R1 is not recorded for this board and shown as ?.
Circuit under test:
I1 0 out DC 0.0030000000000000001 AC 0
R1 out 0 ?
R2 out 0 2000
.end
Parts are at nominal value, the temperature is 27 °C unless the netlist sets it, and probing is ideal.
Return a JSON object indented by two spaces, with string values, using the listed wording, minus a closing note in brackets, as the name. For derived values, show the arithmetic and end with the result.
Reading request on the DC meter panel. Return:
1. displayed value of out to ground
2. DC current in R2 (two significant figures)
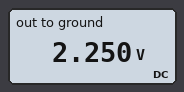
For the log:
{
  "displayed value of out to ground": "2.250 V",
  "DC current in R2": "(2.25 V) / 2 kΩ = 1.1 mA"
}
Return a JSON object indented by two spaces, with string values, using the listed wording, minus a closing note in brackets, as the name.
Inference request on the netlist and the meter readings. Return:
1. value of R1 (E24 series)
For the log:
{
  "value of R1": "1.2 kΩ"
}
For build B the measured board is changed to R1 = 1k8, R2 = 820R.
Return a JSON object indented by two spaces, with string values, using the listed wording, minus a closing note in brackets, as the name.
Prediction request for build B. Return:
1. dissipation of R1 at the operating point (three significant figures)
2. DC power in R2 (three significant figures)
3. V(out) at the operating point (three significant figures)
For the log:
{
  "dissipation of R1 at the operating point": "1.59 mW",
  "DC power in R2": "3.48 mW",
  "V(out) at the operating point": "1.69 V"
}
